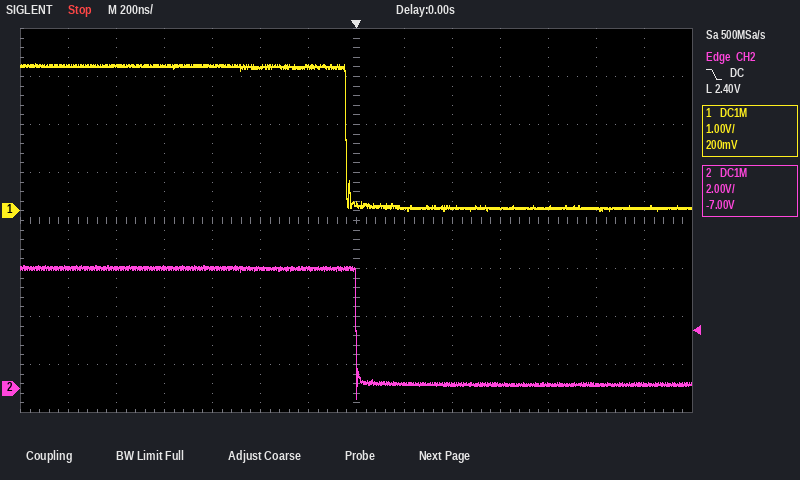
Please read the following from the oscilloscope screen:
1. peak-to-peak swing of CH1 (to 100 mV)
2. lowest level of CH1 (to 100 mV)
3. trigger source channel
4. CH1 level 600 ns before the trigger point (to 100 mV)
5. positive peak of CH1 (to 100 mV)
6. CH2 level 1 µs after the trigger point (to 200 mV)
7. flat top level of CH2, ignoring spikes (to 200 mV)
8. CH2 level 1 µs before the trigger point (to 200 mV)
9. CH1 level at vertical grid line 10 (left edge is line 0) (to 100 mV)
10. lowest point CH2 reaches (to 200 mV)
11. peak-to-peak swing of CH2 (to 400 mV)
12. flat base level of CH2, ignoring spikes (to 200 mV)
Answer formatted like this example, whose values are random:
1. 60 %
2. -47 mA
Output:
1. 3.1 V
2. 0.0 V
3. CH2
4. 3.0 V
5. 3.1 V
6. 200 mV
7. 5.0 V
8. 5.0 V
9. 100 mV
10. -400 mV
11. 5.6 V
12. 200 mV
